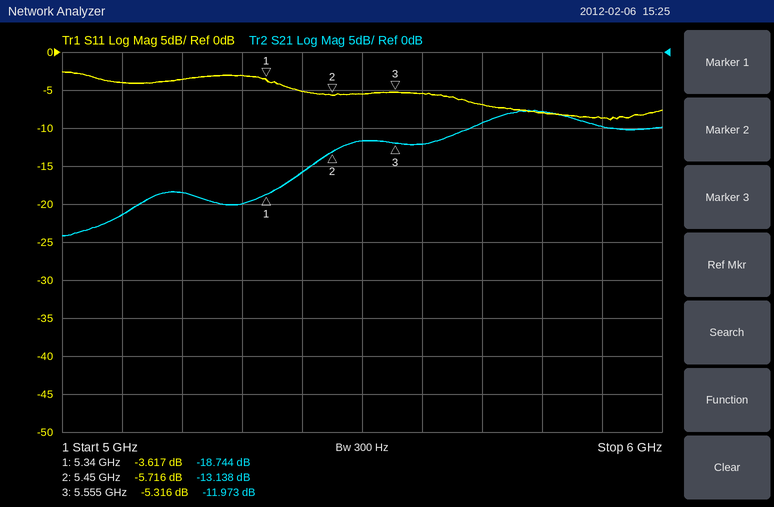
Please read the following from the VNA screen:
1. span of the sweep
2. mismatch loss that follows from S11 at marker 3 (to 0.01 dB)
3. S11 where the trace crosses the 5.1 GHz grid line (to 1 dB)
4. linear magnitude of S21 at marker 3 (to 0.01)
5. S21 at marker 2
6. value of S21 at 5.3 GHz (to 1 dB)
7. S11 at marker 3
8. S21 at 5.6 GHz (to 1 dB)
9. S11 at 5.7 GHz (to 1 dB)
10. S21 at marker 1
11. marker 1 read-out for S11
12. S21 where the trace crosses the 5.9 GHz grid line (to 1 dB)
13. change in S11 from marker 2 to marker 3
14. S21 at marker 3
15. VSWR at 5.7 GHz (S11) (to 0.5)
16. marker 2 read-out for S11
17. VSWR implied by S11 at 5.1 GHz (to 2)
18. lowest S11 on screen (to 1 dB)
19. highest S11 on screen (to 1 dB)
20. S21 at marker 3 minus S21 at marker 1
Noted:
1 GHz
1.51 dB
-4 dB
0.25
-13.138 dB
-20 dB
-5.316 dB
-12 dB
-7 dB
-18.744 dB
-3.617 dB
-10 dB
0.400 dB
-11.973 dB
2.5
-5.716 dB
4
-9 dB
-3 dB
6.771 dB
